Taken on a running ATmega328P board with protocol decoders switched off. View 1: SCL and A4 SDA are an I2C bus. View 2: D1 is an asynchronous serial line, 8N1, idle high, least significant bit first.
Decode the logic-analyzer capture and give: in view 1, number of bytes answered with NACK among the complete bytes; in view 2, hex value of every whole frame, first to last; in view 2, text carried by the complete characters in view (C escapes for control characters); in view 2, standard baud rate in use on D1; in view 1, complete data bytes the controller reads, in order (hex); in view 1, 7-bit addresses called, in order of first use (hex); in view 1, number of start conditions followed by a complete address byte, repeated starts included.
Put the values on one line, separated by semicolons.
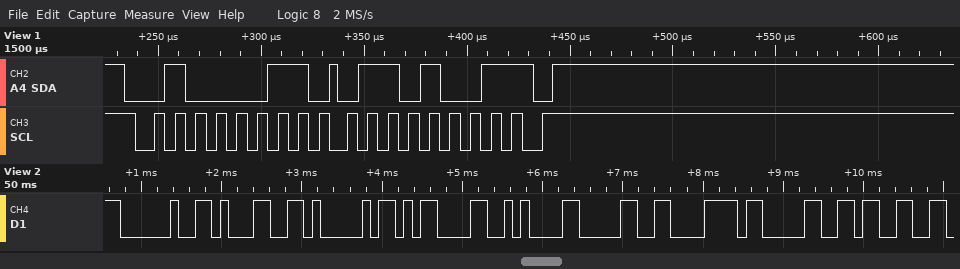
1; 0x20 0x31 0x41 0x0D 0x0A 0x30 0x78 0x30 0x33; " 1A\r\n0x03"; 9600 baud; 69; 0x21; 1
